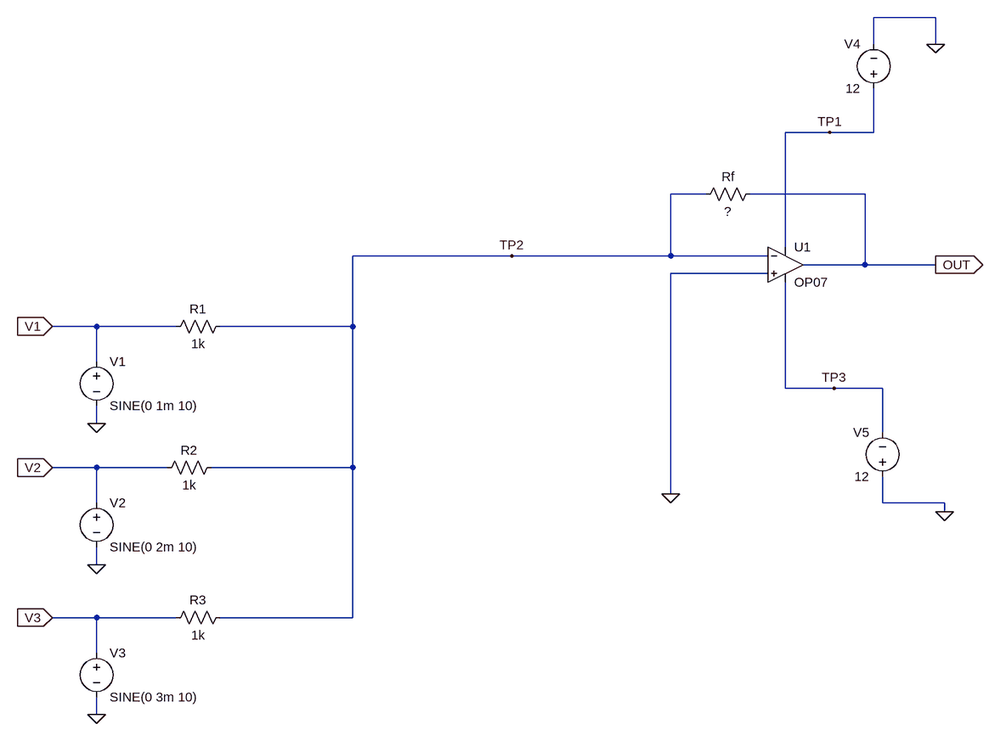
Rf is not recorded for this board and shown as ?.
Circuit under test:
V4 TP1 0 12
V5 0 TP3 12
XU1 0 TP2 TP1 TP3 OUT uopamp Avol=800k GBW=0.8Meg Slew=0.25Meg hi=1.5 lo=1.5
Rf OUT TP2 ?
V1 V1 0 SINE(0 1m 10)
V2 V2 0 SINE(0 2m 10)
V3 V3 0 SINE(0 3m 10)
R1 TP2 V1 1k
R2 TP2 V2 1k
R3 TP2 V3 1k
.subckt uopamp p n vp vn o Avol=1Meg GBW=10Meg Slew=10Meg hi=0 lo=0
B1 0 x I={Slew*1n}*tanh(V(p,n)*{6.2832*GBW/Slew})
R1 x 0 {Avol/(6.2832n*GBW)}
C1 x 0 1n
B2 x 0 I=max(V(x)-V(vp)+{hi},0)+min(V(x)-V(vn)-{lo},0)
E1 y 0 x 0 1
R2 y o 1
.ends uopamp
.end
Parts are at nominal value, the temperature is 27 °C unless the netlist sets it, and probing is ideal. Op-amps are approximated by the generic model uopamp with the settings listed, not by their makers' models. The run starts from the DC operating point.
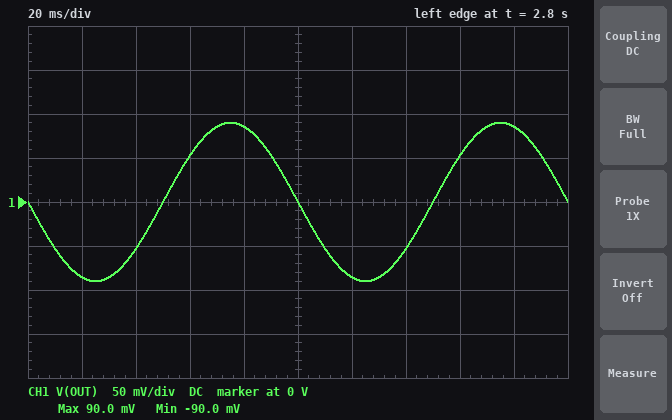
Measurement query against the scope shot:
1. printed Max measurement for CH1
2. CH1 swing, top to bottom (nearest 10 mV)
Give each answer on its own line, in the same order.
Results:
90.0 mV
180 mV
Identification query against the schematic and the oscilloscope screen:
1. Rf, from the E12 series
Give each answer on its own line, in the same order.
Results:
15 kΩ
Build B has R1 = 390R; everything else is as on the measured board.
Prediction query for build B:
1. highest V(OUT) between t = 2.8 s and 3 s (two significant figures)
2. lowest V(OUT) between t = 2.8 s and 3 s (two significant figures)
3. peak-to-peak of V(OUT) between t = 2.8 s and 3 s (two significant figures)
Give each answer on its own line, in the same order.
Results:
110 mV
-110 mV
230 mV
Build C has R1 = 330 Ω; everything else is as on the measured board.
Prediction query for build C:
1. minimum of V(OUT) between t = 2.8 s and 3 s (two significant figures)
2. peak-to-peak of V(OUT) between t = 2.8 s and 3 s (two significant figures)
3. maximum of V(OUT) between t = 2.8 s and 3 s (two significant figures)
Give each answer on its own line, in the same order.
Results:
-120 mV
240 mV
120 mV
